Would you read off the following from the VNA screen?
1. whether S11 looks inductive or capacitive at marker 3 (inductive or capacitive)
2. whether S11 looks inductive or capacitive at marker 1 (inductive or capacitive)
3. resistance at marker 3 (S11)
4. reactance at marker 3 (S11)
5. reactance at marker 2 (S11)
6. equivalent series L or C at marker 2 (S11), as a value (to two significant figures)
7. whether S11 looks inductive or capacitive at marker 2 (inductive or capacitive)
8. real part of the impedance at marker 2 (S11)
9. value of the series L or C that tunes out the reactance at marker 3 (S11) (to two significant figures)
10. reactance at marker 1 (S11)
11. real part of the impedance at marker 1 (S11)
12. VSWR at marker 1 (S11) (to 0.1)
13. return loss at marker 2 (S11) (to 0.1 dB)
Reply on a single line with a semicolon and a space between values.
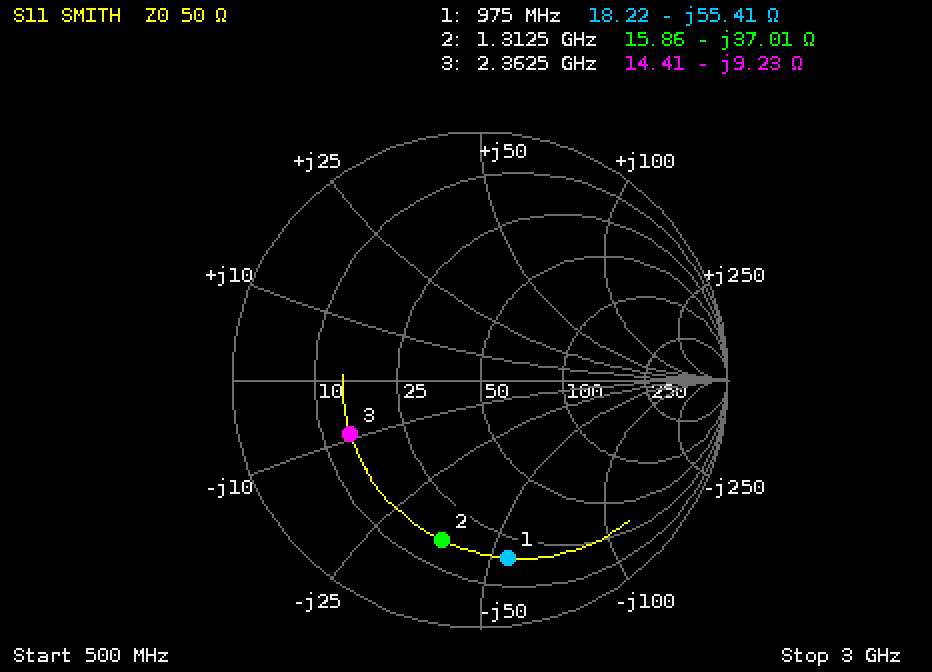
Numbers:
capacitive; capacitive; 14.41 Ω; -9.23 Ω; -37.01 Ω; 3.3 pF; capacitive; 15.86 Ω; 620 pH; -55.41 Ω; 18.22 Ω; 6.3; 3.5 dB
